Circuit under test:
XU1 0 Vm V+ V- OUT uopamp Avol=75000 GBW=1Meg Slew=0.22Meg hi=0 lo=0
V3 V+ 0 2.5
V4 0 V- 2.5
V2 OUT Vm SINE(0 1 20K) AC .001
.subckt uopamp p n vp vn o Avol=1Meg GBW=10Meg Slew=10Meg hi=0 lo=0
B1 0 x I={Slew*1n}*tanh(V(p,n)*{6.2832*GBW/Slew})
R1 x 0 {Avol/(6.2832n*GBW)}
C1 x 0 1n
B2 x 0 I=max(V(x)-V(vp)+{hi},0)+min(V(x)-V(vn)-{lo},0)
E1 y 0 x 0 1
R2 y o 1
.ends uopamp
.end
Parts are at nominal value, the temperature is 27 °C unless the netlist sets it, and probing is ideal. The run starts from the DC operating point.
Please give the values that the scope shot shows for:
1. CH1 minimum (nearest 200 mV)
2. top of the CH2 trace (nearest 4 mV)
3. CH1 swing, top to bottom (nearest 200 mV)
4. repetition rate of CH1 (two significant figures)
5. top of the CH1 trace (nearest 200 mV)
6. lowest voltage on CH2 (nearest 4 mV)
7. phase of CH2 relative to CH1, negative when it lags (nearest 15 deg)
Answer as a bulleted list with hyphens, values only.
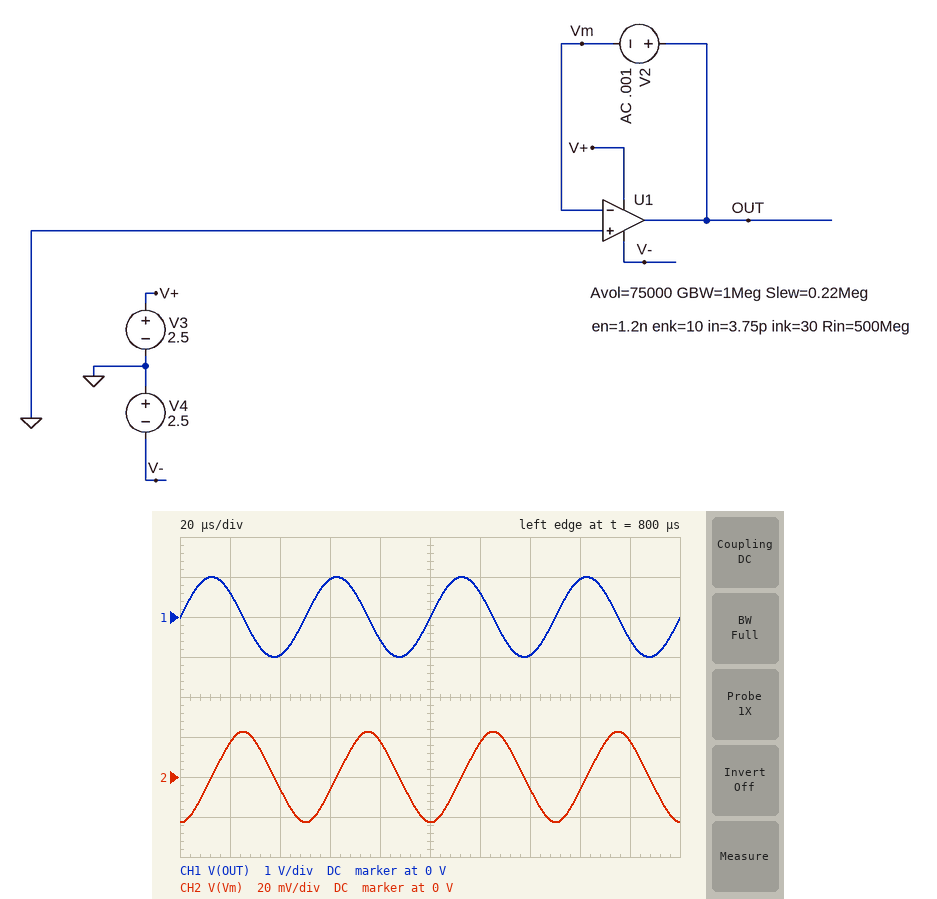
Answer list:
- -1.0 V
- 24 mV
- 2.0 V
- 20 kHz
- 1.0 V
- -24 mV
- -90 deg
